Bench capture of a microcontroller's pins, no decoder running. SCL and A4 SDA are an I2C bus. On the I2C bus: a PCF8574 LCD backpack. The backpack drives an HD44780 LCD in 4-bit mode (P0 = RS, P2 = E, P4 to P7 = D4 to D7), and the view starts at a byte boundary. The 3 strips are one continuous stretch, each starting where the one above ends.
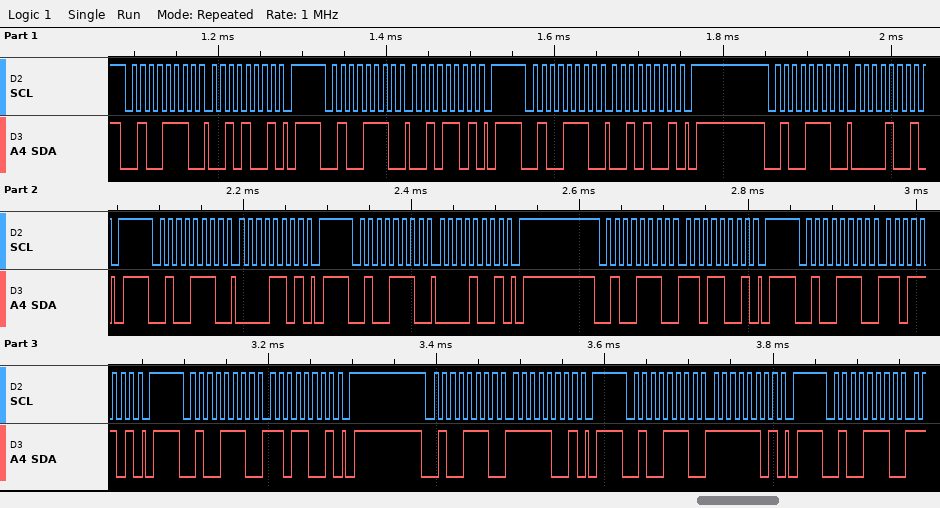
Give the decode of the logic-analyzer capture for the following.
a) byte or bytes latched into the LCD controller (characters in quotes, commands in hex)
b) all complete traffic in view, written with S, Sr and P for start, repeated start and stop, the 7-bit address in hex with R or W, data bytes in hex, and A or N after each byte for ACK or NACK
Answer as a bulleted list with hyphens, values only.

- ' '
- S 27W A 29 A P S 27W A 2D A P S 27W A 29 A P S 27W A 09 A P S 27W A 0D A P S 27W A 09 A P S 27W A D9 A P S 27W A DD A P S 27W A D9 A P S 27W A F9 A P S 27W A FD A P S 27W A
